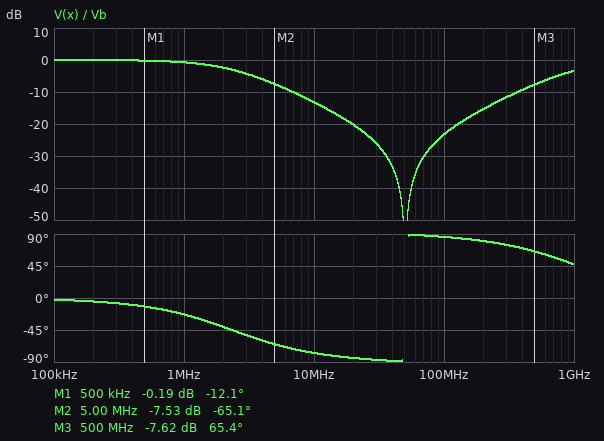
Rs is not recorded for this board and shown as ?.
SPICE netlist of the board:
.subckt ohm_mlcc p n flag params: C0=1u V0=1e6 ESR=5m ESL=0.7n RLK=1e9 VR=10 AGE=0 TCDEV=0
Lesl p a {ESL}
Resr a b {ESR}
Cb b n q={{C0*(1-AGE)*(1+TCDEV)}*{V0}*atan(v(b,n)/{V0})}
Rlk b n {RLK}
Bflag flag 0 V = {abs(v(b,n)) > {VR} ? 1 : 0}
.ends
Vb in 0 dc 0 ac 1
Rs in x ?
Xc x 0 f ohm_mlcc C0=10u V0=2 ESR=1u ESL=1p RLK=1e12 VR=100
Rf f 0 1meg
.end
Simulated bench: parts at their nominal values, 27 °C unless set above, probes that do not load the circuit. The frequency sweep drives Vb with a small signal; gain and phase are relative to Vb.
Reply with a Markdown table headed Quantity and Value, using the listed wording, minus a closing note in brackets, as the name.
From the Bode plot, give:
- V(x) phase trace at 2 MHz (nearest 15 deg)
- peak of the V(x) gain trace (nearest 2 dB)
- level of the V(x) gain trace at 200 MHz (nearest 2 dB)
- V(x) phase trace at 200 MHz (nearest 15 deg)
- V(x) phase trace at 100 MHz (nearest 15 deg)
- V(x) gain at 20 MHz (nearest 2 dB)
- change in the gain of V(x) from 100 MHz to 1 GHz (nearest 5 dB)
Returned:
| Quantity | Value |
|---|---|
| V(x) phase trace at 2 MHz | -45 deg |
| peak of the V(x) gain trace | 0 dB |
| level of the V(x) gain trace at 200 MHz | -16 dB |
| V(x) phase trace at 200 MHz | 75 deg |
| V(x) phase trace at 100 MHz | 90 deg |
| V(x) gain at 20 MHz | -20 dB |
| change in the gain of V(x) from 100 MHz to 1 GHz | 20 dB |
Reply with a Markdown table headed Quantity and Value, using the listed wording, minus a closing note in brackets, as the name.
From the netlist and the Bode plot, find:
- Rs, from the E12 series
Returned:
| Quantity | Value |
|---|---|
| Rs, from the E12 series | 6.8 mΩ |
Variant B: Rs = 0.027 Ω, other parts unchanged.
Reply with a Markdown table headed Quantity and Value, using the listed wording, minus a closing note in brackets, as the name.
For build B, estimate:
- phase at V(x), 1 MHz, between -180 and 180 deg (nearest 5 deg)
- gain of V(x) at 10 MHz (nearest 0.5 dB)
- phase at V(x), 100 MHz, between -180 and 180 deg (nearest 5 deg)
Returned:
| Quantity | Value |
|---|---|
| phase at V(x), 1 MHz, between -180 and 180 deg | -60 deg |
| gain of V(x) at 10 MHz | -25.0 dB |
| phase at V(x), 100 MHz, between -180 and 180 deg | 90 deg |
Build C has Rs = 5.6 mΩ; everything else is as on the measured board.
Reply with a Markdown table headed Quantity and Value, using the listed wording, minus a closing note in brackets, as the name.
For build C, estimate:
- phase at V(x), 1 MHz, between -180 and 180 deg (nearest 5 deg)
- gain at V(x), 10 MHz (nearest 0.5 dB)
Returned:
| Quantity | Value |
|---|---|
| phase at V(x), 1 MHz, between -180 and 180 deg | -20 deg |
| gain at V(x), 10 MHz | -11.5 dB |
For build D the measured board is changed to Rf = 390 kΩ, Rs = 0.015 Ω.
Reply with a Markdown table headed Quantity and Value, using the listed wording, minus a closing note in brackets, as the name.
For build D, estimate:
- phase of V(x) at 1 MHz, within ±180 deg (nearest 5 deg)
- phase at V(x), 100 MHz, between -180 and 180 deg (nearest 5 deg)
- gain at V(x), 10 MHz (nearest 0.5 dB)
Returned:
| Quantity | Value |
|---|---|
| phase of V(x) at 1 MHz, within ±180 deg | -45 deg |
| phase at V(x), 100 MHz, between -180 and 180 deg | 90 deg |
| gain at V(x), 10 MHz | -20.0 dB |
